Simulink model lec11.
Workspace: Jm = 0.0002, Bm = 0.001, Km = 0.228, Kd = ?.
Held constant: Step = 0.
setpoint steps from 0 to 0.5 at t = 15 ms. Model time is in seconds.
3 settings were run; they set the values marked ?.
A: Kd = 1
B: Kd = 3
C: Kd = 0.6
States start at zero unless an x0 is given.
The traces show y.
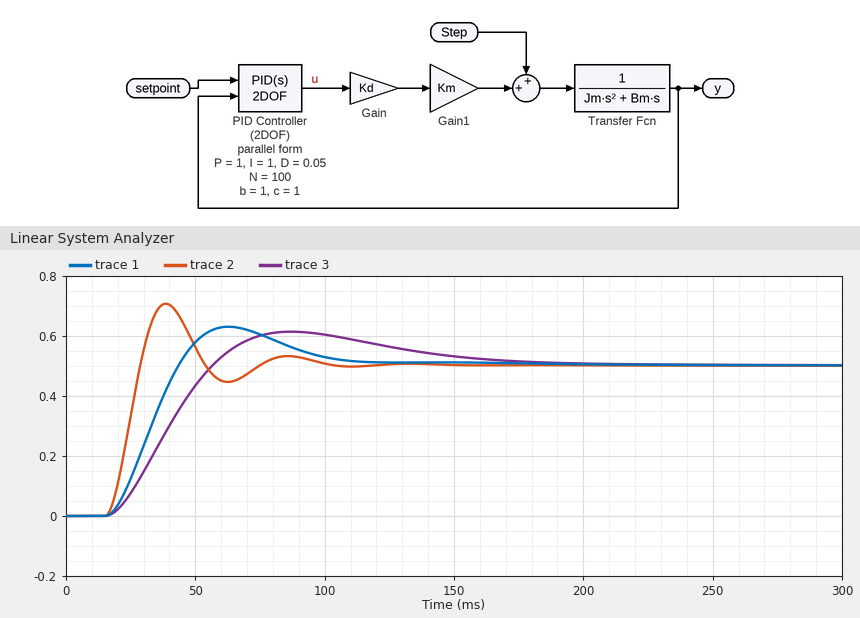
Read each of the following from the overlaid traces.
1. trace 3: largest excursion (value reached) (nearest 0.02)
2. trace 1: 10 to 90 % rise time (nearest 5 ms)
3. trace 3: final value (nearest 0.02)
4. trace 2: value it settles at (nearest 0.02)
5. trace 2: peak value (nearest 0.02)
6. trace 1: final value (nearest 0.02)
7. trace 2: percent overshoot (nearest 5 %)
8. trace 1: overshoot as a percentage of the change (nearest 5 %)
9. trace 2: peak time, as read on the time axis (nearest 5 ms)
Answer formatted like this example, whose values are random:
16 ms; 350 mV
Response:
0.62; 20 ms; 0.50; 0.50; 0.70; 0.50; 40 %; 25 %; 40 ms
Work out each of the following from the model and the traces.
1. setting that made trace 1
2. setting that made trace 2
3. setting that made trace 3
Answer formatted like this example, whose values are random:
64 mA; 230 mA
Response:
A; B; C
